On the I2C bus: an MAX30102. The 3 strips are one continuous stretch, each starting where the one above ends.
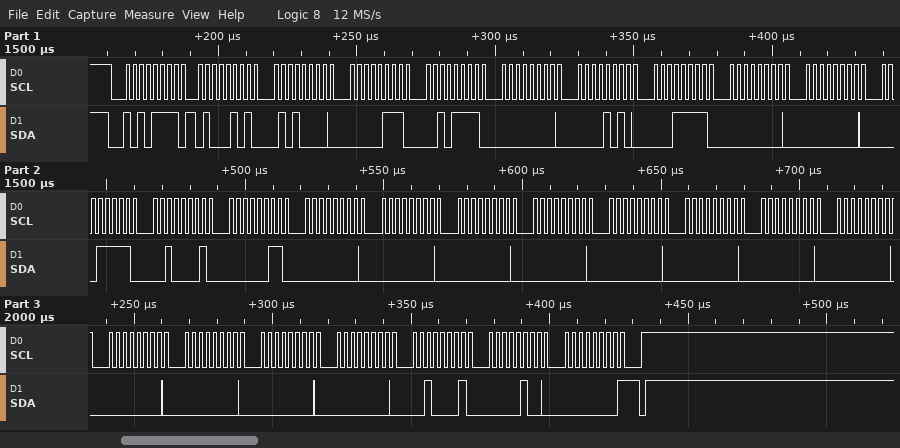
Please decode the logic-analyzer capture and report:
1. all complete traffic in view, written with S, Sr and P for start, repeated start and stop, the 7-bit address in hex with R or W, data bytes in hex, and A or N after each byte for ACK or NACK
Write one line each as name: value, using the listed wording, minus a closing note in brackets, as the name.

all complete traffic in view, written with S, Sr and P for start, repeated start and stop, the 7-bit address in hex with R or W, data bytes in hex, and A or N after each byte for ACK or NACK: S 57R A 45 A 50 A 07 A 2F A 00 A 0A A 1F A 00 A 00 A 1F A 21 A 03 A 00 A 00 A 00 A 00 A 00 A 00 A 00 A 00 A 00 A 00 A 00 A 00 A 21 A 04 A 00 N P
